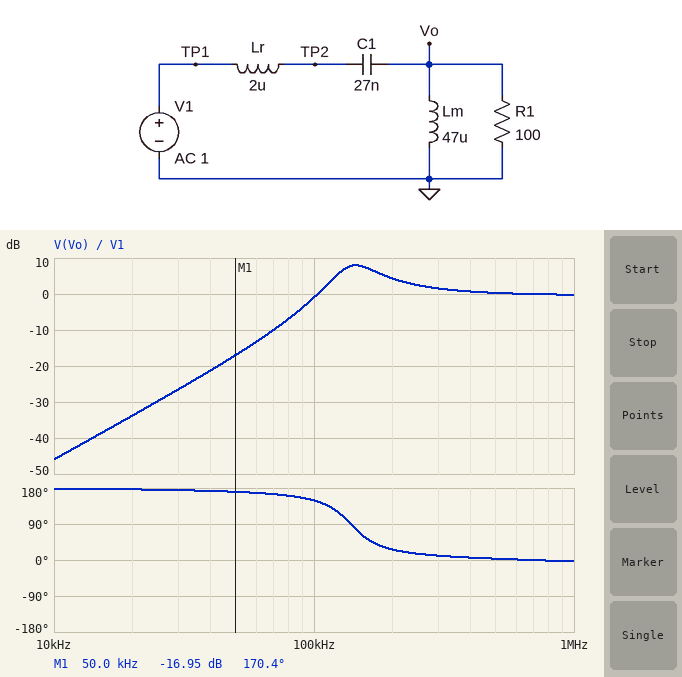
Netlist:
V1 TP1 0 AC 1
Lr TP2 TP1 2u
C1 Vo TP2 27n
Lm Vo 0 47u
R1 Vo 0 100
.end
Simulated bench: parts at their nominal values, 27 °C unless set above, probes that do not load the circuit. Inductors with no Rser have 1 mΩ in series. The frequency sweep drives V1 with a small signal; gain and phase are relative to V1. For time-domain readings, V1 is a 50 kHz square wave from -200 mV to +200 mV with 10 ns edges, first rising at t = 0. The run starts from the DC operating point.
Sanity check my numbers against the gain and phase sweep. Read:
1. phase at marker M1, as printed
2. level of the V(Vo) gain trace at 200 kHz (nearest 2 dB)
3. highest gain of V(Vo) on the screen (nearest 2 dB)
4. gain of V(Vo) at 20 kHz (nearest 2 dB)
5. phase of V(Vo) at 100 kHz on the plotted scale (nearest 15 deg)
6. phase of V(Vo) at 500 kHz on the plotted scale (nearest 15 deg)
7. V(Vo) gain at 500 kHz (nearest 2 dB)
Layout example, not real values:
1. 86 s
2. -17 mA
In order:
1. 170.4 deg
2. 4 dB
3. 8 dB
4. -34 dB
5. 150 deg
6. 0 deg
7. 0 dB
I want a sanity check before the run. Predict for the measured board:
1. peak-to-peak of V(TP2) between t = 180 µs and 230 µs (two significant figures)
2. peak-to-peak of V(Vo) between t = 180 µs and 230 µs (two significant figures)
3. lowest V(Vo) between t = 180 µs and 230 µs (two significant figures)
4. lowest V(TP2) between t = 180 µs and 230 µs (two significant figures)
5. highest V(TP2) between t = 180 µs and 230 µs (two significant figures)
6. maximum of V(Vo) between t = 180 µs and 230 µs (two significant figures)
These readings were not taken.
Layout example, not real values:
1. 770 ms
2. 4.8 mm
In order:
1. 420 mV
2. 860 mV
3. -430 mV
4. -210 mV
5. 210 mV
6. 430 mV
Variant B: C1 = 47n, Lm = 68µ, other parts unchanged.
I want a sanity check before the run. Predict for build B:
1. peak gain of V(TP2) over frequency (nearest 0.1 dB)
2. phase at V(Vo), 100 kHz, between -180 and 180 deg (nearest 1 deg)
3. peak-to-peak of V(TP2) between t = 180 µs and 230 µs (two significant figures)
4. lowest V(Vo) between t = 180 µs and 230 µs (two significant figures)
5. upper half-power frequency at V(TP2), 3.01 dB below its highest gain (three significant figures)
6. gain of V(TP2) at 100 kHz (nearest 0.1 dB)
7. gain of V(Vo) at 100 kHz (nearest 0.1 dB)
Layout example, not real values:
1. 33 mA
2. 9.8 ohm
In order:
1. 0.4 dB
2. 54 deg
3. 410 mV
4. -280 mV
5. 6.96 MHz
6. -0.1 dB
7. 7.9 dB
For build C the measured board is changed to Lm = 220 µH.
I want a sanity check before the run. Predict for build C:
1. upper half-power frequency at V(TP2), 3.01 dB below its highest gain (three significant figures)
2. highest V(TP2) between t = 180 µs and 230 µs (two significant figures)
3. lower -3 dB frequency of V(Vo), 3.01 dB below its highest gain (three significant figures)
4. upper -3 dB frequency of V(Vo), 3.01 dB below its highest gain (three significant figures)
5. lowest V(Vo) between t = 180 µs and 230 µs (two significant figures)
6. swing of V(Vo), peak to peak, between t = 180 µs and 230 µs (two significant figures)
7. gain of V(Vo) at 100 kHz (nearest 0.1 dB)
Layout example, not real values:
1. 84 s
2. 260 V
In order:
1. 7.80 MHz
2. 200 mV
3. 55.1 kHz
4. 4.21 MHz
5. -420 mV
6. 850 mV
7. 1.7 dB
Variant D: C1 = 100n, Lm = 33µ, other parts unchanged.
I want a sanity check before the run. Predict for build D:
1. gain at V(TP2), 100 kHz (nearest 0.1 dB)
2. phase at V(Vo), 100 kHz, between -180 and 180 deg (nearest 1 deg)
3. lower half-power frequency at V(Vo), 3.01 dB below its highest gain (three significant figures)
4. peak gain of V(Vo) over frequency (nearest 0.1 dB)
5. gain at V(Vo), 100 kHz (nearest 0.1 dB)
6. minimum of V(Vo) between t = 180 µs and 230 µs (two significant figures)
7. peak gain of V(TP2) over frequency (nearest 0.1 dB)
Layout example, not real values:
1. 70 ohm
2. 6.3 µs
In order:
1. -1.3 dB
2. 27 deg
3. 79.3 kHz
4. 15.1 dB
5. 9.7 dB
6. -230 mV
7. 1.6 dB
